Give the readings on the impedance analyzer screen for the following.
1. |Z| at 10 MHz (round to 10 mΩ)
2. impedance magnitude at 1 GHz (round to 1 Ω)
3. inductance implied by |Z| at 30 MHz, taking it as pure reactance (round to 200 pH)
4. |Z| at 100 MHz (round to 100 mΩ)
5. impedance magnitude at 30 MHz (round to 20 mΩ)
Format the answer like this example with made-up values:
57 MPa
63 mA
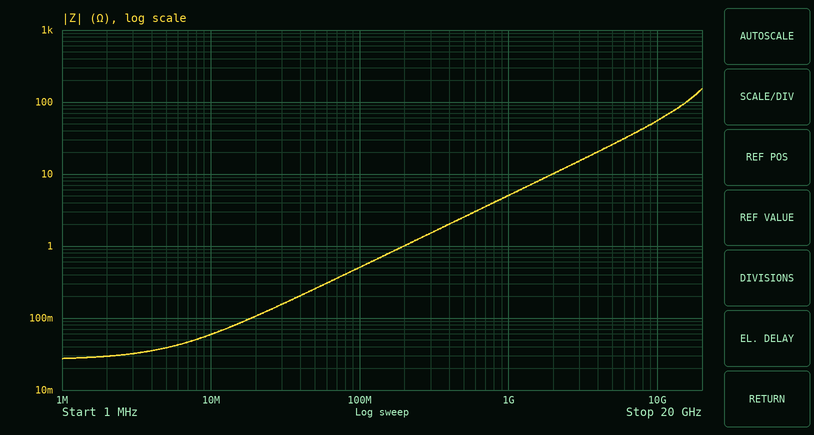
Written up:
60 mΩ
5 Ω
800 pH
500 mΩ
160 mΩ
